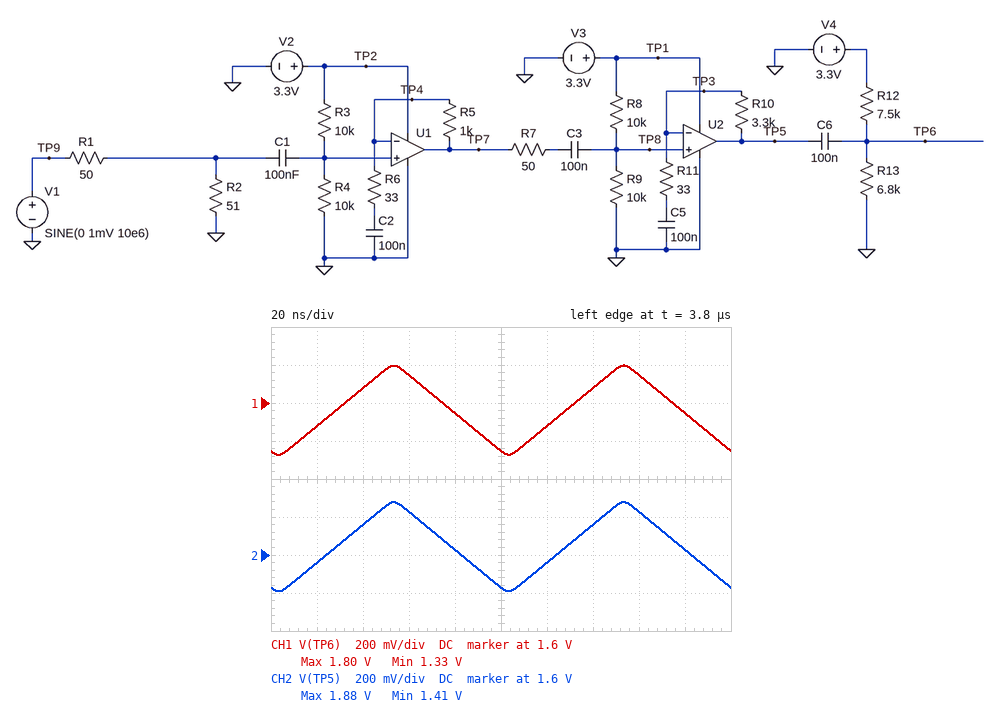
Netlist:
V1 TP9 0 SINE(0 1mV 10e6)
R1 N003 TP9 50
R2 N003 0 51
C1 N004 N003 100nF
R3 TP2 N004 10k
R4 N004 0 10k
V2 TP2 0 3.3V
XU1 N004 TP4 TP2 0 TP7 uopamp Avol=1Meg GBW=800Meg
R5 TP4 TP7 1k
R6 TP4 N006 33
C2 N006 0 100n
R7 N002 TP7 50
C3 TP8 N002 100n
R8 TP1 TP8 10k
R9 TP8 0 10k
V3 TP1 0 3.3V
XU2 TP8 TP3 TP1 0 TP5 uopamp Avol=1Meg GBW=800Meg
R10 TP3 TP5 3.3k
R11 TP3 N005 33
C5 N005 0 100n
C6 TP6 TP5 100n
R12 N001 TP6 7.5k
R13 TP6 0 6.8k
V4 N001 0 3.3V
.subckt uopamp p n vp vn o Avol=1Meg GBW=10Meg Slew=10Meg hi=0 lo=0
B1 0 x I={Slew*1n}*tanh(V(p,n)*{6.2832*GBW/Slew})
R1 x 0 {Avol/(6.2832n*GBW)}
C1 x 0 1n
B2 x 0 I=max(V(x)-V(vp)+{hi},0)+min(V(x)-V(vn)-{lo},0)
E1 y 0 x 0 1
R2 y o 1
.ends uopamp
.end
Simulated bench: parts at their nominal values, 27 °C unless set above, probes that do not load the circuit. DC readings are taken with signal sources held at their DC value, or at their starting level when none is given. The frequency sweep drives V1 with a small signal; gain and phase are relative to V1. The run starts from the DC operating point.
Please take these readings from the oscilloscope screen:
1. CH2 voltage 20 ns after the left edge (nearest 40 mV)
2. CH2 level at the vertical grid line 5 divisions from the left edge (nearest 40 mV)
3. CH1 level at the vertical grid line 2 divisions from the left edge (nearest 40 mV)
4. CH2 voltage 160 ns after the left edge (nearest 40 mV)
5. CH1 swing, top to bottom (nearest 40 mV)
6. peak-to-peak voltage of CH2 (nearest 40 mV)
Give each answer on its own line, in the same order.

1.56 V
1.44 V
1.68 V
1.84 V
480 mV
480 mV
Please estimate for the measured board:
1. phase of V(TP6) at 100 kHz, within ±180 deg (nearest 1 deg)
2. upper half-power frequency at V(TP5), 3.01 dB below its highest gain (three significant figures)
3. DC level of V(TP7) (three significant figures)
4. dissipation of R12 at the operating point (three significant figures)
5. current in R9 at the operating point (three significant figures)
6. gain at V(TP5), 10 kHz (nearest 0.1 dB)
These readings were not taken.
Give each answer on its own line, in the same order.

50 deg
7.38 MHz
1.65 V
399 µW
165 µA
36.3 dB
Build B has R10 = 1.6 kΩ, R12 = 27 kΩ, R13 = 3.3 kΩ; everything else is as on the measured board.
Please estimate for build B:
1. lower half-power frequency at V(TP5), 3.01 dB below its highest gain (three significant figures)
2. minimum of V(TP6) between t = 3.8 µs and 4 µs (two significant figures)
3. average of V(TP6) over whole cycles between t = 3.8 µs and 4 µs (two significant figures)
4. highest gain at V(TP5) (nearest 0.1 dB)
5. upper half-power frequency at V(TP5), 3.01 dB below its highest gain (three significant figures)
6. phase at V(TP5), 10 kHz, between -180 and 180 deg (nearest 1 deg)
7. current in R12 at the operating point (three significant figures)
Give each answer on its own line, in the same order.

74.4 kHz
120 mV
360 mV
57.7 dB
12.7 MHz
146 deg
109 µA
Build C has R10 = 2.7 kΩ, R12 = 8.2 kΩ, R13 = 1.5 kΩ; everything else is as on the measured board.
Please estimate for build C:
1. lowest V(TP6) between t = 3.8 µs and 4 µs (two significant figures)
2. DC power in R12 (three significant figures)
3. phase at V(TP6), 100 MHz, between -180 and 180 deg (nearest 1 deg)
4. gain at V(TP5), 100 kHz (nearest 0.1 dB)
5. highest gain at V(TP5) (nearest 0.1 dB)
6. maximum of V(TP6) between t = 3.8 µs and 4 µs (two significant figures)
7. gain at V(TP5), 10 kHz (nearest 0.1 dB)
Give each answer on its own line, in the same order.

270 mV
949 µW
-160 deg
60.4 dB
62.2 dB
740 mV
34.6 dB
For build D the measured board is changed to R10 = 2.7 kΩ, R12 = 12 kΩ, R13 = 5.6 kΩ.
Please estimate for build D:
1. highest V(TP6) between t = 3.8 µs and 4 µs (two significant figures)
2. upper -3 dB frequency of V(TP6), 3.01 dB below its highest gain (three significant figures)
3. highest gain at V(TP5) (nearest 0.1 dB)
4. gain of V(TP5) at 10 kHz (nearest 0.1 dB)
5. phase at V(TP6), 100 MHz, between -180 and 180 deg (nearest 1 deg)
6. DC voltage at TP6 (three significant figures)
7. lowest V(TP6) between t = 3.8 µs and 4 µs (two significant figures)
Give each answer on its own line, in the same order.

1.3 V
8.69 MHz
62.2 dB
34.6 dB
-160 deg
1.05 V
810 mV
